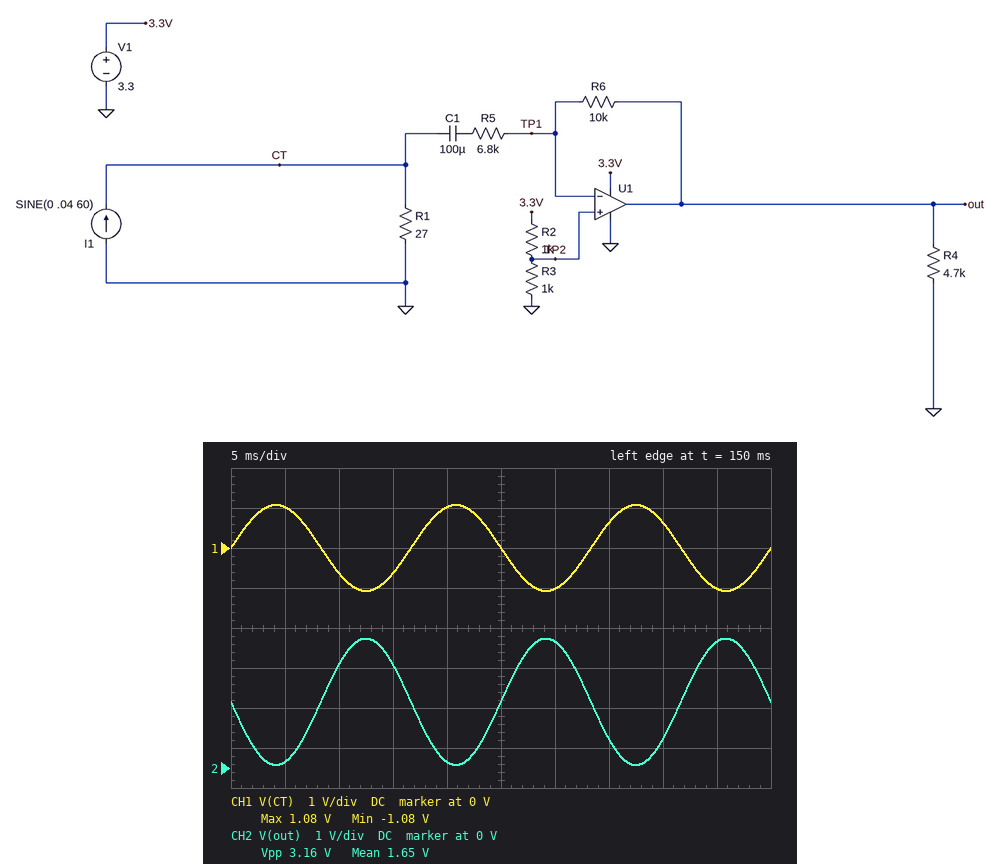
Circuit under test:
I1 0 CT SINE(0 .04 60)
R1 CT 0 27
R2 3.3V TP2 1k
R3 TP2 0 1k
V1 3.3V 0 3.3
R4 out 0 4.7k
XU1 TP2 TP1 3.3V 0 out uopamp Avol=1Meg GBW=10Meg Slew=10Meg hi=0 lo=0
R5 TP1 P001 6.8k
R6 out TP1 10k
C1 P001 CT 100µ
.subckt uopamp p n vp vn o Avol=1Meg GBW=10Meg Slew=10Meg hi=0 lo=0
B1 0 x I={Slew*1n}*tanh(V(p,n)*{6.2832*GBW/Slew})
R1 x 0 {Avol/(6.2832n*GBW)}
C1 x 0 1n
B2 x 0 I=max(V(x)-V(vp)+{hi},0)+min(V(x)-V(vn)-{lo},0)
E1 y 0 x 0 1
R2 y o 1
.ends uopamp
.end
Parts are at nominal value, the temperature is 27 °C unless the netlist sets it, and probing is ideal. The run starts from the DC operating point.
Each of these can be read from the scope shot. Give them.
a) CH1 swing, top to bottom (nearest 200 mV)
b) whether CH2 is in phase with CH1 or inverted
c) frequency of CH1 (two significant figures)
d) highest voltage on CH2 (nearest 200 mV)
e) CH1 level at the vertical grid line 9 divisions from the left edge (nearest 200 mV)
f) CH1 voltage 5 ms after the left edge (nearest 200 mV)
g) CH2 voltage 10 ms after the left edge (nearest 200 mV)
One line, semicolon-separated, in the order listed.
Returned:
2.2 V; inverted; 60 Hz; 3.2 V; -1.0 V; 1.0 V; 2.6 V
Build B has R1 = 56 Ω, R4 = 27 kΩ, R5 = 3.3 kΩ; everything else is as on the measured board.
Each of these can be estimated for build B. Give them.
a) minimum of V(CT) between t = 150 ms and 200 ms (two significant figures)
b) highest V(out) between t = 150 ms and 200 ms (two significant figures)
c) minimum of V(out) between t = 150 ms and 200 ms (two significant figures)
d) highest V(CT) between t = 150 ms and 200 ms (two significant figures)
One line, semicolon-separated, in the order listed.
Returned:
-2.2 V; 3.3 V; -9.8 mV; 2.2 V
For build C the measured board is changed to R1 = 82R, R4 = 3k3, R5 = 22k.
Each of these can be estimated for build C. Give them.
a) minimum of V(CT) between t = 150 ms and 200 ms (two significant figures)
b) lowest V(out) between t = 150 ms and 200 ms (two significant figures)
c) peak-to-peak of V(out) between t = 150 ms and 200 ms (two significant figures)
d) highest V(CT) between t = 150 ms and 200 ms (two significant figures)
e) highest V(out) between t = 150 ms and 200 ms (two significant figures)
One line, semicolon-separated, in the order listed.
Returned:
-3.3 V; 170 mV; 3.0 V; 3.3 V; 3.1 V
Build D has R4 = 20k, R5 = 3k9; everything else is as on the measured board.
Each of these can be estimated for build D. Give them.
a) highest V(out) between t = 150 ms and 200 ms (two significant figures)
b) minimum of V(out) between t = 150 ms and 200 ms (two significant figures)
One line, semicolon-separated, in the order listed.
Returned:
3.3 V; -9.4 mV
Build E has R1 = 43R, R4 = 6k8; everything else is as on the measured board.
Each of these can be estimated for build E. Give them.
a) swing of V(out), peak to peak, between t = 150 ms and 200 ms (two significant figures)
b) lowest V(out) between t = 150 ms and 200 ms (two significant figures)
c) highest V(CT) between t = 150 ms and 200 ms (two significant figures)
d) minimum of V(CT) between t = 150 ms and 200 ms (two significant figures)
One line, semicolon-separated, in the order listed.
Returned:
3.3 V; -9.5 mV; 1.7 V; -1.7 V
